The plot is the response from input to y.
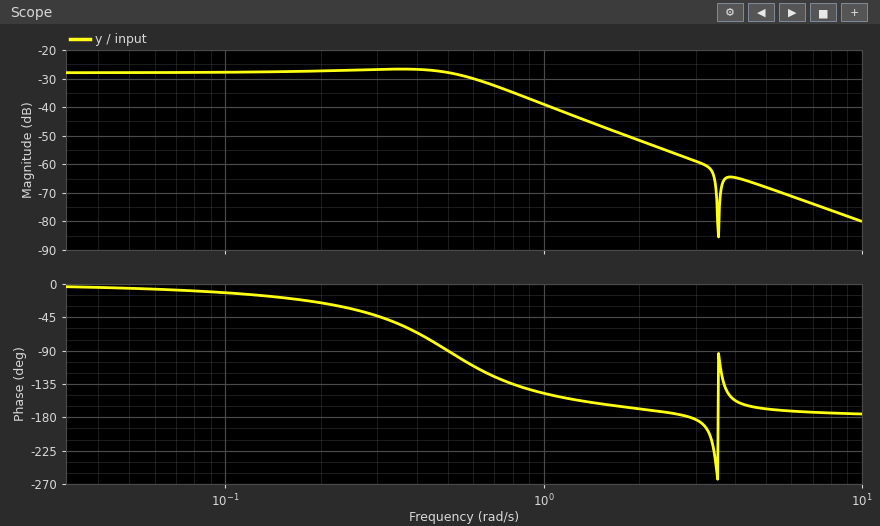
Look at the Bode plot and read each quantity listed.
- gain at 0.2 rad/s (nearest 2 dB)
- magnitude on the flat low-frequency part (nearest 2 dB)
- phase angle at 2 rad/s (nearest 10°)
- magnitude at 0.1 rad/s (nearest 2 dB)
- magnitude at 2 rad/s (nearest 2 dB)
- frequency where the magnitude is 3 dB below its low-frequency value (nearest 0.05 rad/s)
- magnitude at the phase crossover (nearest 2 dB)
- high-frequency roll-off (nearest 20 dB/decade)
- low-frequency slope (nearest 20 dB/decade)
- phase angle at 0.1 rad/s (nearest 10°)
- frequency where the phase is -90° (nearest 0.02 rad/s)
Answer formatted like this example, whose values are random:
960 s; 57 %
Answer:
-28 dB; -28 dB; -170°; -28 dB; -52 dB; 0.65 rad/s; -58 dB; -40 dB/decade; 0 dB/decade; -10°; 0.50 rad/s
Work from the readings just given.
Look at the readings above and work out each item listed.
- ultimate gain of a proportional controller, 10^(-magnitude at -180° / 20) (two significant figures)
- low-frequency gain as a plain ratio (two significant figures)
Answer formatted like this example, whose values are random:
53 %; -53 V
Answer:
790; 0.040
